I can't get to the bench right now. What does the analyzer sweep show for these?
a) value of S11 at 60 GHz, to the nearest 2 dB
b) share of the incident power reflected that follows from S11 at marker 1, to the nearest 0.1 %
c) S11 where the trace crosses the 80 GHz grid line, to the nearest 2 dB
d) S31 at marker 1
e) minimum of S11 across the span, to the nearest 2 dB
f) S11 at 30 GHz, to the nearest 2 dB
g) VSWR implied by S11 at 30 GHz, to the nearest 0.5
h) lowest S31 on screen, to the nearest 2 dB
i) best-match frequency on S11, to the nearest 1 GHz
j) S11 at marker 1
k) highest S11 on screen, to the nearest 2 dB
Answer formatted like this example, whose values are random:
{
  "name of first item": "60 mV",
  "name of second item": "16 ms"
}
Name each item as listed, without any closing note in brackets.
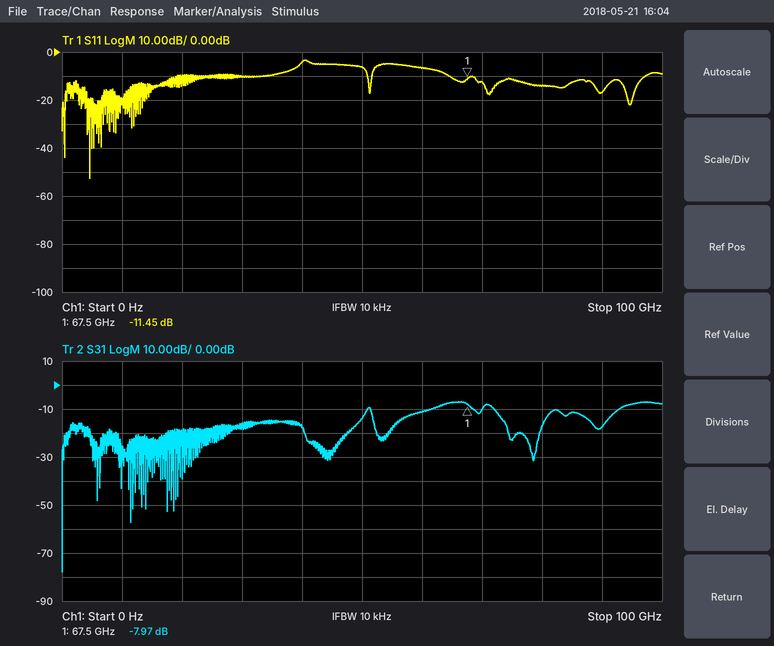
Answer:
{
  "value of S11 at 60 GHz, to the nearest 2 dB": "-6 dB",
  "share of the incident power reflected that follows from S11 at marker 1, to the nearest 0.1 %": "7.2 %",
  "S11 where the trace crosses the 80 GHz grid line, to the nearest 2 dB": "-14 dB",
  "S31 at marker 1": "-7.97 dB",
  "minimum of S11 across the span, to the nearest 2 dB": "-52 dB",
  "S11 at 30 GHz, to the nearest 2 dB": "-10 dB",
  "VSWR implied by S11 at 30 GHz, to the nearest 0.5": "2.0",
  "lowest S31 on screen, to the nearest 2 dB": "-78 dB",
  "best-match frequency on S11, to the nearest 1 GHz": "5 GHz",
  "S11 at marker 1": "-11.45 dB",
  "highest S11 on screen, to the nearest 2 dB": "-4 dB"
}
